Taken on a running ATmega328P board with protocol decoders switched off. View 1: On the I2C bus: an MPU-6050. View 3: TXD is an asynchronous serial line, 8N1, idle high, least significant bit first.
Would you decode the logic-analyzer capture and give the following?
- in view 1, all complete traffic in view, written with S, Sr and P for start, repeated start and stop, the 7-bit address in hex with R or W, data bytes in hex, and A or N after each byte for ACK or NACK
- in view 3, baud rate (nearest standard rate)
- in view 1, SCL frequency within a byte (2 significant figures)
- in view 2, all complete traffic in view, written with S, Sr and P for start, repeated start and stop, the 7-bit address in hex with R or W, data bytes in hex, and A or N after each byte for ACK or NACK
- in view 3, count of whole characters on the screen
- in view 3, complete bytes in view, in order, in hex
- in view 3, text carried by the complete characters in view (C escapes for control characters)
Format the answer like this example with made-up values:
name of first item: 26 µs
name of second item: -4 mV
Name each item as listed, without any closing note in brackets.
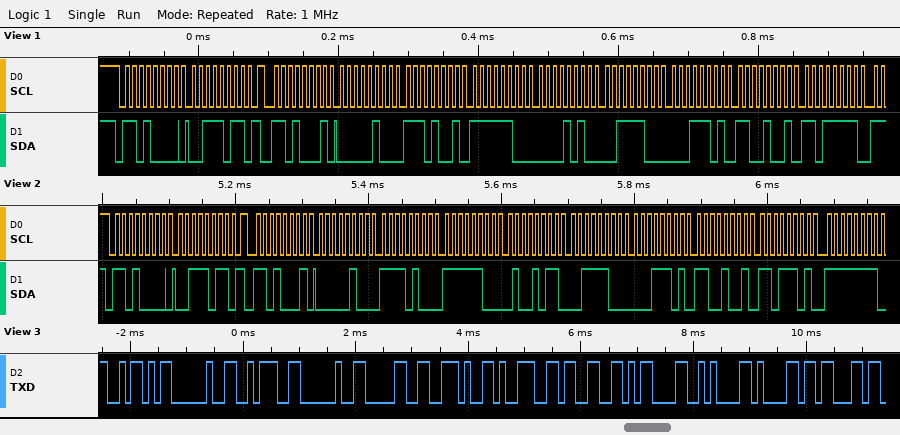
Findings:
in view 1, all complete traffic in view, written with S, Sr and P for start, repeated start and stop, the 7-bit address in hex with R or W, data bytes in hex, and A or N after each byte for ACK or NACK: S 68W A 3B A Sr 68R A 04 A E9 A FC A 0A A 3C A 1D A C9 A DF A
in view 3, baud rate: 9600 baud
in view 1, SCL frequency within a byte: 100 kHz
in view 2, all complete traffic in view, written with S, Sr and P for start, repeated start and stop, the 7-bit address in hex with R or W, data bytes in hex, and A or N after each byte for ACK or NACK: S 68W A 3B A Sr 68R A 04 A F4 A FC A 4B A 3C A 1D A C9 A DD A FF A
in view 3, count of whole characters on the screen: 12
in view 3, complete bytes in view, in order, in hex: 5A 20 3A 20 30 2E 39 33 0D 0A 61 63
in view 3, text carried by the complete characters in view: "Z : 0.93\r\nac"
